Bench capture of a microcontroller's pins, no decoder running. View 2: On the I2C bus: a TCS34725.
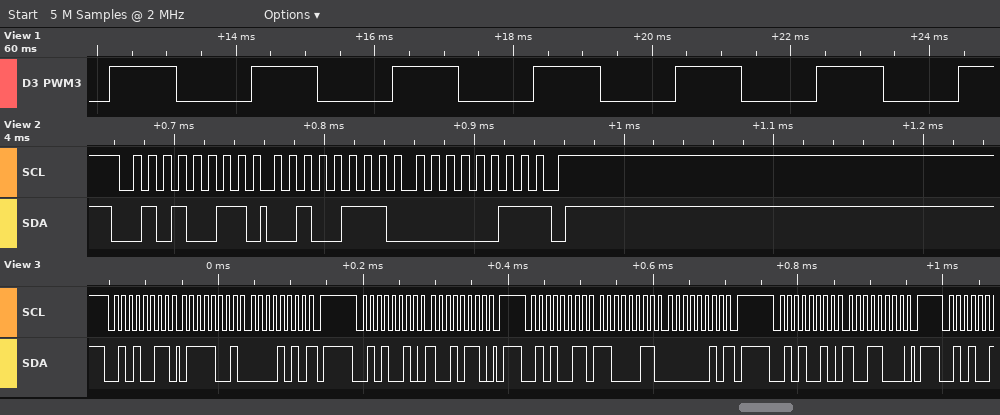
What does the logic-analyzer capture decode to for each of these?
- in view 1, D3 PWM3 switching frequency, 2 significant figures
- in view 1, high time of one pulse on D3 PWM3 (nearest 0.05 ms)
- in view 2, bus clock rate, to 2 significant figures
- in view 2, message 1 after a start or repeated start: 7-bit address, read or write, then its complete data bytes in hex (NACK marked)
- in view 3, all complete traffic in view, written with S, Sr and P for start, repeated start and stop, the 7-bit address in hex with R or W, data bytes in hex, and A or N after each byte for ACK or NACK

490 Hz
0.95 ms
100 kHz
0x29 read: 27 03 NACK
S 29R A 79 A 0A N P S 29W A 96 A P S 29R A C3 A 02 N P S 29W A 98 A P
